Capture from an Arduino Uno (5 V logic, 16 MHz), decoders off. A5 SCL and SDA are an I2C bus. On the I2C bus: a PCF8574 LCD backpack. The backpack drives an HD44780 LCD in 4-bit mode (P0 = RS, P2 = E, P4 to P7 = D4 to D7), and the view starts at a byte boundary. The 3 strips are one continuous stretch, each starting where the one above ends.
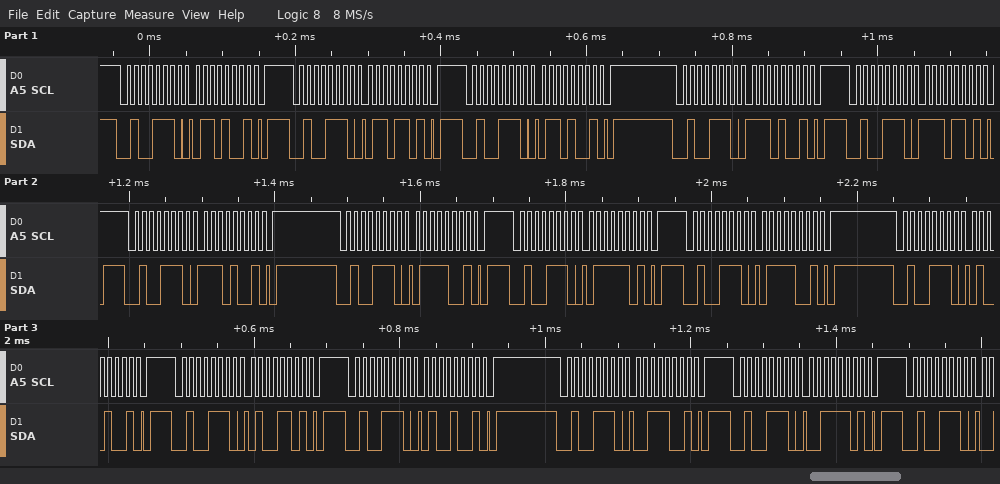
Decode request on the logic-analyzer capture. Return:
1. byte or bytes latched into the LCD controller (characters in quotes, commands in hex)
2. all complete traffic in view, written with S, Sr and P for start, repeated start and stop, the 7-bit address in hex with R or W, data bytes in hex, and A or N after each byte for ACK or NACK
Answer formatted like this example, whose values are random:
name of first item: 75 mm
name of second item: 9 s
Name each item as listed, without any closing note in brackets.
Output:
byte or bytes latched into the LCD controller: 'n' 't'
all complete traffic in view, written with S, Sr and P for start, repeated start and stop, the 7-bit address in hex with R or W, data bytes in hex, and A or N after each byte for ACK or NACK: S 27W A 69 A P S 27W A 6D A P S 27W A 69 A P S 27W A E9 A P S 27W A ED A P S 27W A E9 A P S 27W A 79 A P S 27W A 7D A P S 27W A 79 A P S 27W A 49 A P S 27W A 4D A P S 27W A 49 A P S 27W A 39 A P S 27W A 3D A P S 27W A
